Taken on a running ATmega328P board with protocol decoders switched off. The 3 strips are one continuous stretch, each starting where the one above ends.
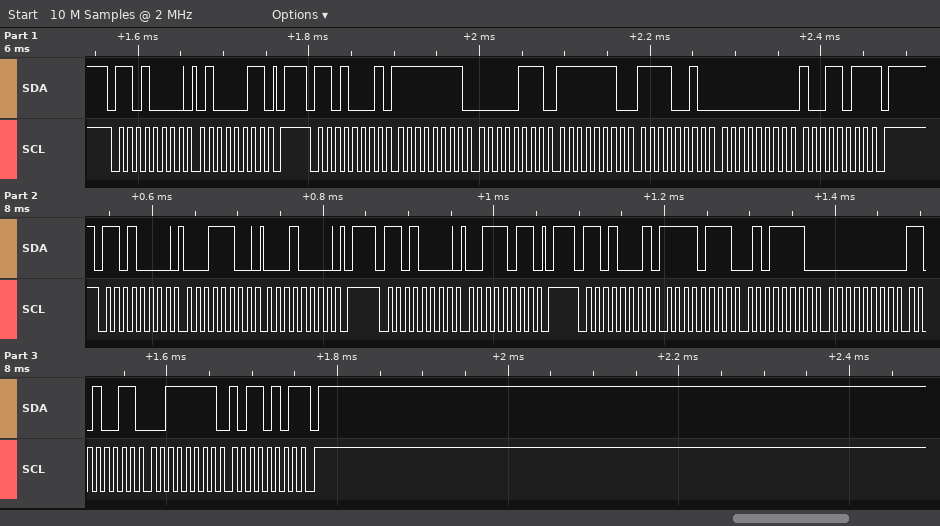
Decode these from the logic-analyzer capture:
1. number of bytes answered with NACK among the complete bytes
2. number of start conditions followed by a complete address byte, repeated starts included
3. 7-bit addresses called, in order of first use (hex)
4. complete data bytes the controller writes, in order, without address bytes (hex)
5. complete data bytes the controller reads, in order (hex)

2
5
0x68
43 1C 10 3B
FF 07 FE F2 00 9B F7 5E 00 D3 3F B5
